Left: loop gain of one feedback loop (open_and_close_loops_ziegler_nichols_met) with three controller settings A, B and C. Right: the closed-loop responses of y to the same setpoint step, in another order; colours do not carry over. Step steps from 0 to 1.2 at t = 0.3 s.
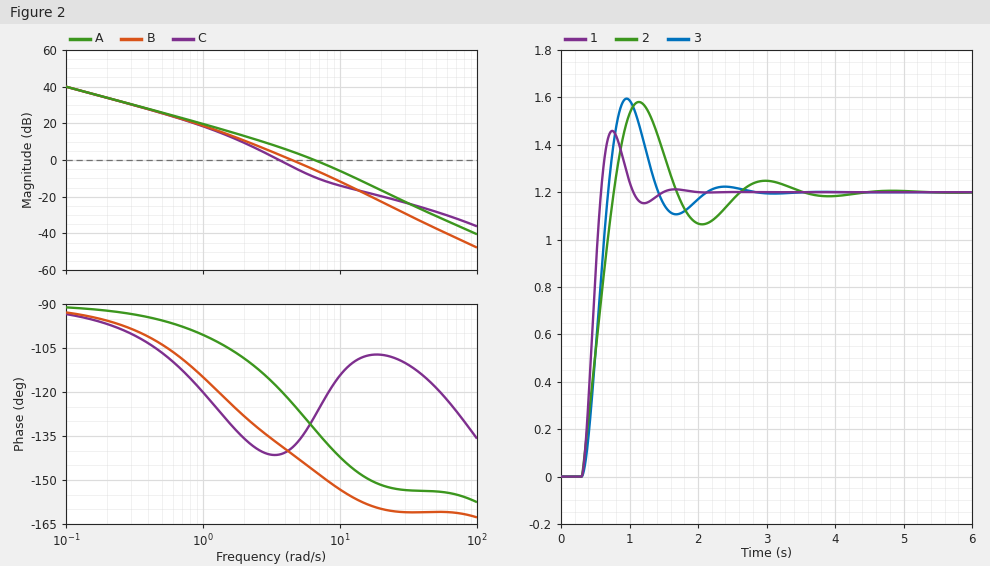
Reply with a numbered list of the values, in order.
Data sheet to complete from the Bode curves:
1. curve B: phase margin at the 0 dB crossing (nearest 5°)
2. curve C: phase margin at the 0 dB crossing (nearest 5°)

1. 40°
2. 40°
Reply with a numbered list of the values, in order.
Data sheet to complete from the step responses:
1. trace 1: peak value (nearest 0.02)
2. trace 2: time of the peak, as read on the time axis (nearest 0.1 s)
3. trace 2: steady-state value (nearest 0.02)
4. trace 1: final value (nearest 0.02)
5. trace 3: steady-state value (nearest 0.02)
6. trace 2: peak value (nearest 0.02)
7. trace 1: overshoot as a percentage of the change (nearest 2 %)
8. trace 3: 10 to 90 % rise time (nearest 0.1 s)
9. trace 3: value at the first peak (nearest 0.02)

1. 1.46
2. 1.1 s
3. 1.20
4. 1.20
5. 1.20
6. 1.58
7. 22 %
8. 0.3 s
9. 1.60
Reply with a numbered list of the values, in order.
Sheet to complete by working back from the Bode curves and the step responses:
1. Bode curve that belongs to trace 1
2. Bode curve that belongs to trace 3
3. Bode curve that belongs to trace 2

1. A
2. B
3. C
